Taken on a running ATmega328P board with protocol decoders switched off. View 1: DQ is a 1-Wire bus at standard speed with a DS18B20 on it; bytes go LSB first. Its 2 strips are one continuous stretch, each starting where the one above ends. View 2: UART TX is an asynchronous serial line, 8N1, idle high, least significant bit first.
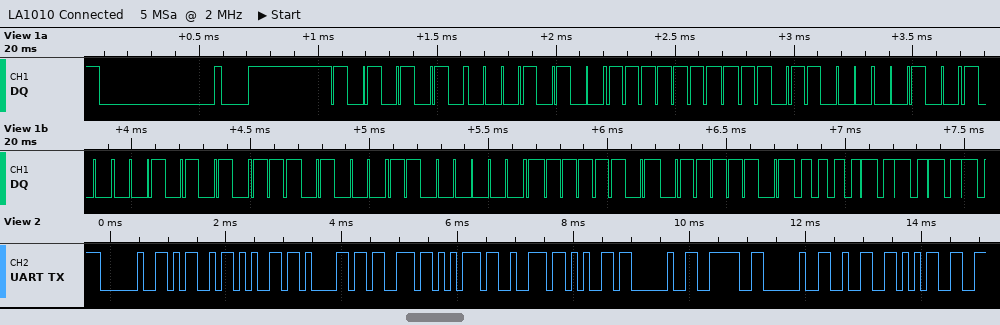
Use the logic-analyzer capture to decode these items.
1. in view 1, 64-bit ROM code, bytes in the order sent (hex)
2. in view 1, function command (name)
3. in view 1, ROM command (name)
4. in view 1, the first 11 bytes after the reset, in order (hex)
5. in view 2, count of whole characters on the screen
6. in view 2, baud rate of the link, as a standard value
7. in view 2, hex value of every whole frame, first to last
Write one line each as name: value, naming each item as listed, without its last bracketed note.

in view 1, 64-bit ROM code, bytes in the order sent: 28 FF 1B 24 54 17 03 BF
in view 1, function command: Read Scratchpad
in view 1, ROM command: Match ROM
in view 1, the first 11 bytes after the reset, in order: 55 28 FF 1B 24 54 17 03 BF BE 50
in view 2, count of whole characters on the screen: 13
in view 2, baud rate of the link, as a standard value: 9600 baud
in view 2, hex value of every whole frame, first to last: 20 4D 65 61 73 75 72 65 20 3E 20 32 35
